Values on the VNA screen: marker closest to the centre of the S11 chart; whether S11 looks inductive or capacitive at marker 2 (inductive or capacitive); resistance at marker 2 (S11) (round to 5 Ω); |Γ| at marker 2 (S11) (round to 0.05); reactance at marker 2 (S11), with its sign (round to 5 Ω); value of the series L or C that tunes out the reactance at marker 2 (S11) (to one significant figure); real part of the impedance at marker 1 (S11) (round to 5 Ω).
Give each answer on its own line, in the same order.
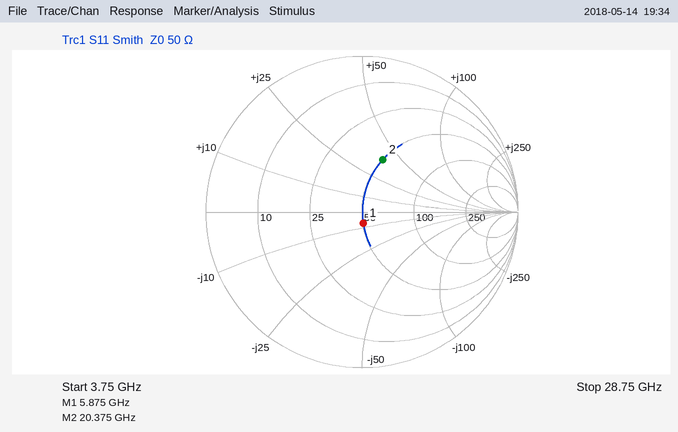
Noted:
marker 1
inductive
50 Ω
0.35
+40 Ω
200 fF
50 Ω
